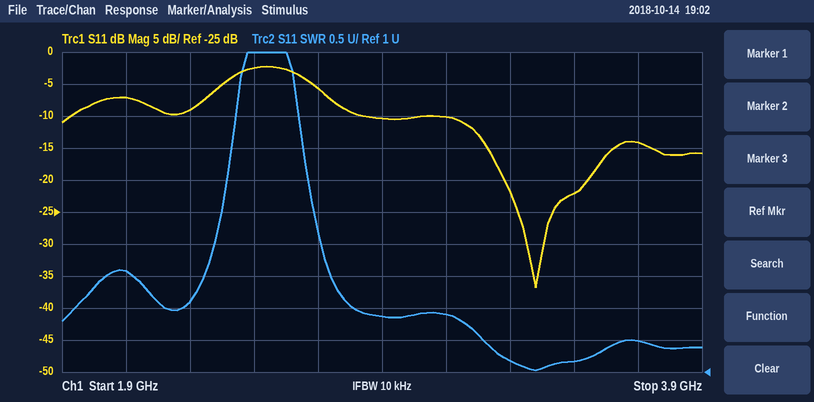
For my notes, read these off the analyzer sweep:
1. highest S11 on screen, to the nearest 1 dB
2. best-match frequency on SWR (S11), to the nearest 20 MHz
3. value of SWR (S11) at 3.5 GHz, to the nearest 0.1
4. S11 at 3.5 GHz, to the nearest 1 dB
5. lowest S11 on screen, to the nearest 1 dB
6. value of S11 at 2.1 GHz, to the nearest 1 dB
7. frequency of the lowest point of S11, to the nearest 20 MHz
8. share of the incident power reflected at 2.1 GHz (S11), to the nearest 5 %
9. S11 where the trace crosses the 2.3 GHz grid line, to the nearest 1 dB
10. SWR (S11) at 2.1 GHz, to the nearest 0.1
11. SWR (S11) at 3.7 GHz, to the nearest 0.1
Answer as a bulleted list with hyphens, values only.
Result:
- -2 dB
- 3.38 GHz
- 1.2
- -22 dB
- -37 dB
- -7 dB
- 3.38 GHz
- 20 %
- -9 dB
- 2.6
- 1.5
